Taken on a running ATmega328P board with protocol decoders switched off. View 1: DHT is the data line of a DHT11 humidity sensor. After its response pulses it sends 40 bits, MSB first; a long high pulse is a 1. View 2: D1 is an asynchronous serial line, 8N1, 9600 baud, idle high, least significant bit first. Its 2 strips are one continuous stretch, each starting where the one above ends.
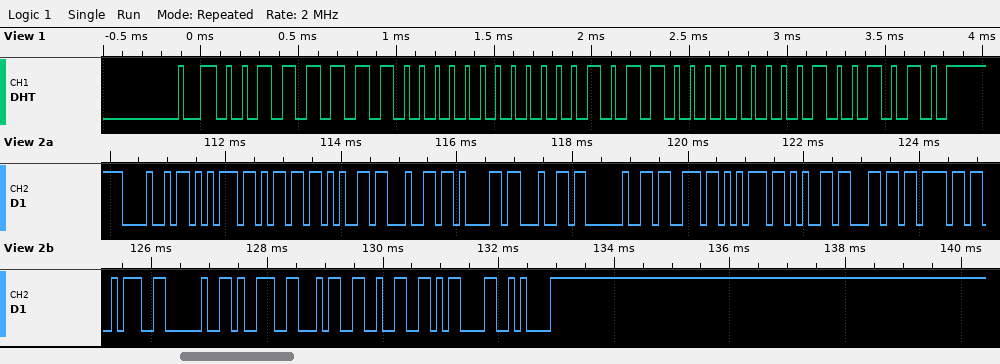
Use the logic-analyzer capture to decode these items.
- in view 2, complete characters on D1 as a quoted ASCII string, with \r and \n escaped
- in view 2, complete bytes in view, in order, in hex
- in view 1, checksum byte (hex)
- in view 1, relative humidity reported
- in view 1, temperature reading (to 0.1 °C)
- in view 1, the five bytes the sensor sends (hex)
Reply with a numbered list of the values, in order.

1. "Humedad suelo: 942\r\n"
2. 48 75 6D 65 64 61 64 20 73 75 65 6C 6F 3A 20 39 34 32 0D 0A
3. 0x4A
4. 63 %
5. 11.0 °C
6. 3F 00 0B 00 4A
